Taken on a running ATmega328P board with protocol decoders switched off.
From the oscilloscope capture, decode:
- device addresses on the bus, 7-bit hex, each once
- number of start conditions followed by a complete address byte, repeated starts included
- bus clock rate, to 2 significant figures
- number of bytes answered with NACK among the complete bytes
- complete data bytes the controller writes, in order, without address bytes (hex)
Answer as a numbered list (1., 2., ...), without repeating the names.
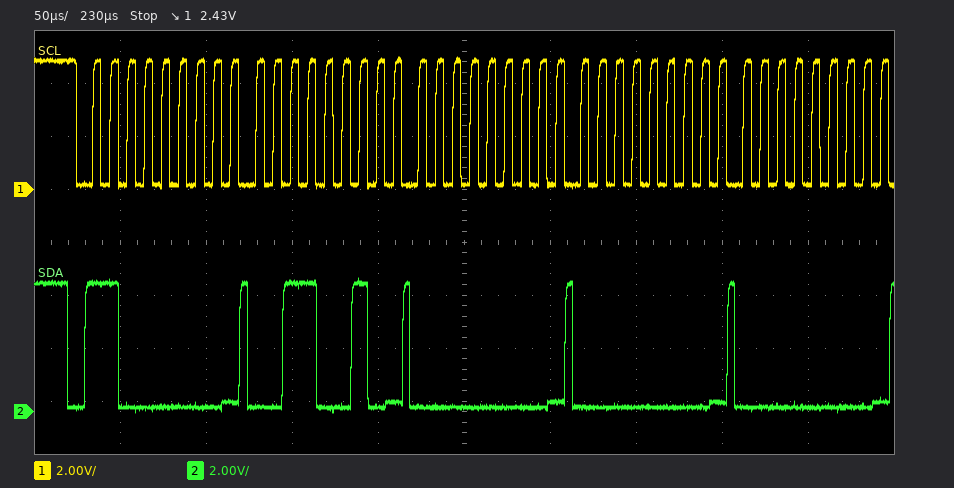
1. 0x60
2. 1
3. 100 kHz
4. 0
5. 32 00 00 00
